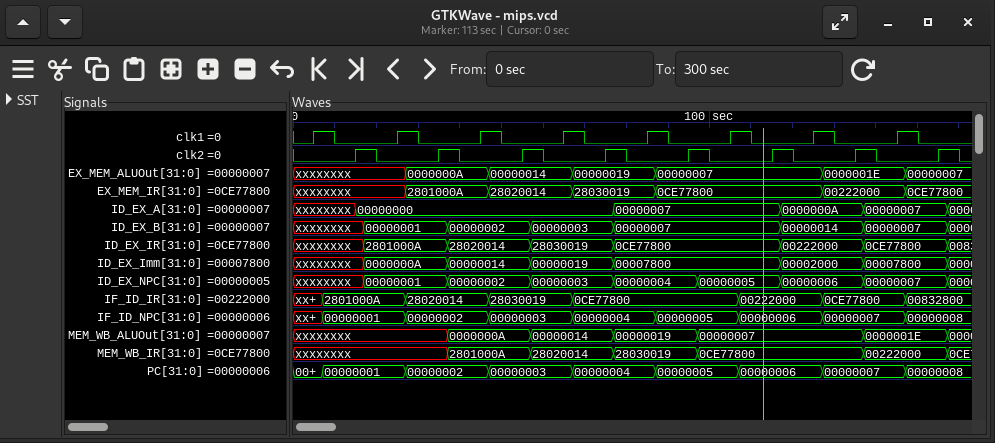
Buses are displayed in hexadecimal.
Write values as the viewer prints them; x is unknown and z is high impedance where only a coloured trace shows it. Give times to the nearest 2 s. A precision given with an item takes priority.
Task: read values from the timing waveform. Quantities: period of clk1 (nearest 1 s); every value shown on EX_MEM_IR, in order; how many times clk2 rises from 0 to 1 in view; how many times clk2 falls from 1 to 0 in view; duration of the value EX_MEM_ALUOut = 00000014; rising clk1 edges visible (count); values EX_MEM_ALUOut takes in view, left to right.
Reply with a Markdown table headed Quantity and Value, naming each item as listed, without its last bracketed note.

| Quantity | Value |
|---|---|
| period of clk1 | 20 s |
| every value shown on EX_MEM_IR, in order | xxxxxxxx, 2801000A, 28020014, 28030019, 0CE77800, 00222000, 0CE77800 |
| how many times clk2 rises from 0 to 1 in view | 8 |
| how many times clk2 falls from 1 to 0 in view | 8 |
| duration of the value EX_MEM_ALUOut = 00000014 | 20 s |
| rising clk1 edges visible | 8 |
| values EX_MEM_ALUOut takes in view, left to right | xxxxxxxx, 0000000A, 00000014, 00000019, 00000007, 0000001E, 00000007 |
